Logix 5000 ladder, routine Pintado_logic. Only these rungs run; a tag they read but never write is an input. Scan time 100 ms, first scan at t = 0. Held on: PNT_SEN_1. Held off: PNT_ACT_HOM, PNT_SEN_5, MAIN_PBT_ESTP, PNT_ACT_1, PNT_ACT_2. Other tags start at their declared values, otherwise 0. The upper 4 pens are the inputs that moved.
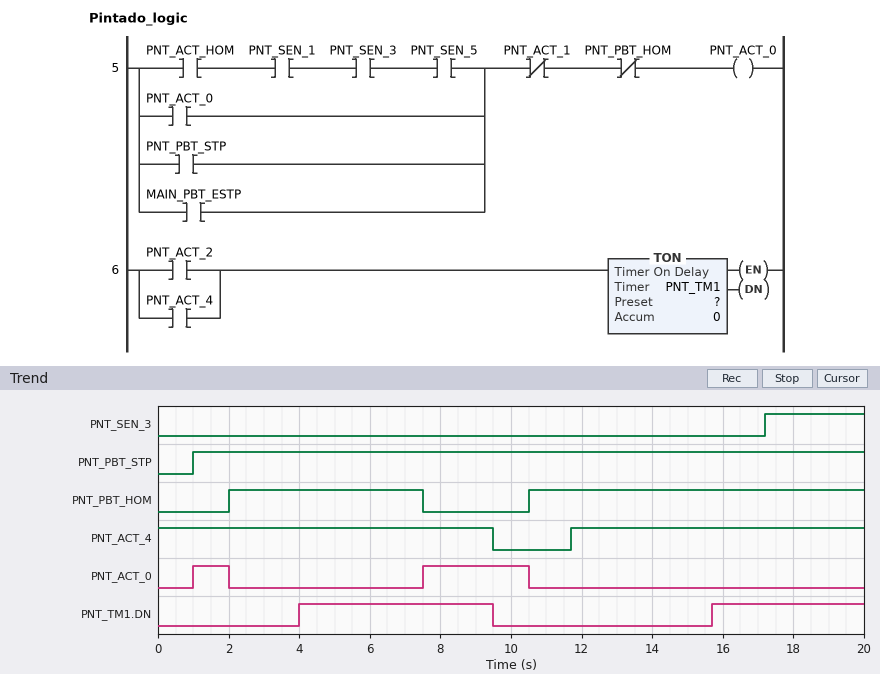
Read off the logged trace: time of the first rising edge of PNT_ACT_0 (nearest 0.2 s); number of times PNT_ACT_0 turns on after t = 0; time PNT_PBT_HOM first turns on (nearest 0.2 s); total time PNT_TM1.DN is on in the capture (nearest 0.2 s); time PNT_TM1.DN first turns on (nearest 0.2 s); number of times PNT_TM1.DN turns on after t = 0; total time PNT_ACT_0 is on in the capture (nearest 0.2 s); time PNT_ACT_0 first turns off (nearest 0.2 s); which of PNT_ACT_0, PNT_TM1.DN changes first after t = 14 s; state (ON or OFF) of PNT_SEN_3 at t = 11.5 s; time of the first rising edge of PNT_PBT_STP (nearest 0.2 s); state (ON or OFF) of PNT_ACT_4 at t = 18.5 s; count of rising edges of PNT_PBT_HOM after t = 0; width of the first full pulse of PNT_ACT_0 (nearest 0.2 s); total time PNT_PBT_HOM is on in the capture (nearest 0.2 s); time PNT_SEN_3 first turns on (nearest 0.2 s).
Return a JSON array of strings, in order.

["1.0 s", "2", "2.0 s", "9.8 s", "4.0 s", "2", "4.0 s", "2.0 s", "PNT_TM1.DN", "OFF", "1.0 s", "ON", "2", "1.0 s", "15.0 s", "17.2 s"]
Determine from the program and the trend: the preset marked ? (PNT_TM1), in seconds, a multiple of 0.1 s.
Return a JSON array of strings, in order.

["4.0 s"]
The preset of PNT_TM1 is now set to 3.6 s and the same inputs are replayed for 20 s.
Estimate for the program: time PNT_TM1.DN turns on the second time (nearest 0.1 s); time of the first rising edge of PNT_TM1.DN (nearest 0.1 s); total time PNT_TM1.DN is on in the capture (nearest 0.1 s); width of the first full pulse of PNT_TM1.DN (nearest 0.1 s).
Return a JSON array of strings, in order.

["15.3 s", "3.6 s", "10.6 s", "5.9 s"]
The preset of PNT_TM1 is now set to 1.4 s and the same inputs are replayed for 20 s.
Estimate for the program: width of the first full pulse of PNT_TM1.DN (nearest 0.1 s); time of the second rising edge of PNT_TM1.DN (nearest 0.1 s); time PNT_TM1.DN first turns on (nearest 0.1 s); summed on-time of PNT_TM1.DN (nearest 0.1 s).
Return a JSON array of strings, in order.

["8.1 s", "13.1 s", "1.4 s", "15.0 s"]
